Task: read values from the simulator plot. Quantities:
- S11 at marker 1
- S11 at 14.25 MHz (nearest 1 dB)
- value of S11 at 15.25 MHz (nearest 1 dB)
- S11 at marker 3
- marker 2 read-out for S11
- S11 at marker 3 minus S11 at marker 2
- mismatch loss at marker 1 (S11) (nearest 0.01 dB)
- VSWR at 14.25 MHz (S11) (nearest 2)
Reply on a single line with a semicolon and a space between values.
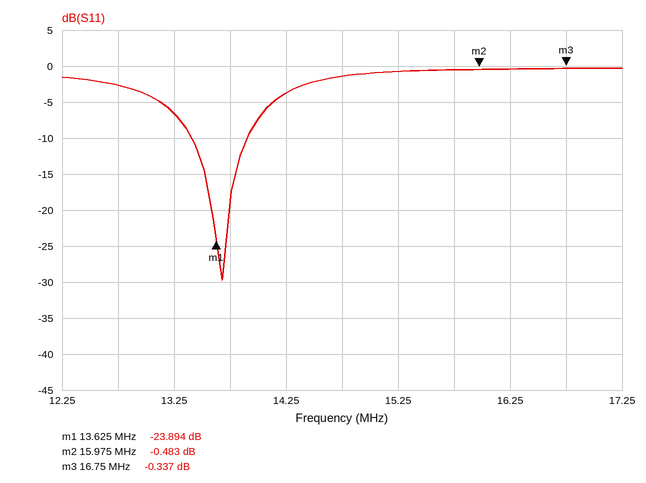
-23.894 dB; -4 dB; -1 dB; -0.337 dB; -0.483 dB; 0.146 dB; 0.02 dB; 4
